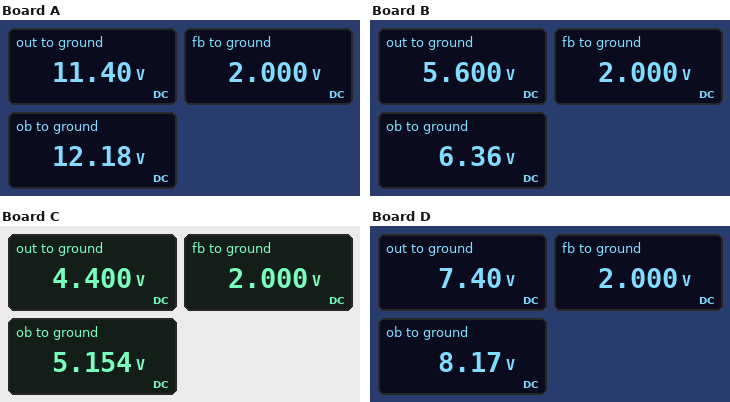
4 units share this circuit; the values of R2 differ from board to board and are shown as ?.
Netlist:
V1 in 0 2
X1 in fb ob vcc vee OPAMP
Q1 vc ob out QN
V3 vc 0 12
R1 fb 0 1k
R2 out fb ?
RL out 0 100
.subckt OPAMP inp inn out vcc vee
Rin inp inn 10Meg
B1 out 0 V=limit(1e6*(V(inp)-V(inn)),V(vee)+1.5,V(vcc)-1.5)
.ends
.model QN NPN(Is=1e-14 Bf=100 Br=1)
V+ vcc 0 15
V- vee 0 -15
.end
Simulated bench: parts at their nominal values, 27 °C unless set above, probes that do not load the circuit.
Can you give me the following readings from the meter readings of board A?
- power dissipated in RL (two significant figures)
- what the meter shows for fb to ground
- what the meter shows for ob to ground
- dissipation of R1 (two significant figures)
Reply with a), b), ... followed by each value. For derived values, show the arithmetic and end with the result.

a) (11.4 V)^2 / 100 Ω = 1.3 W
b) 2.000 V
c) 12.18 V
d) (2 V)^2 / 1 kΩ = 4.0 mW
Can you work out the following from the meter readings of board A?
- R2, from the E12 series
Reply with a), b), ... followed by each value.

a) 4.7 kΩ
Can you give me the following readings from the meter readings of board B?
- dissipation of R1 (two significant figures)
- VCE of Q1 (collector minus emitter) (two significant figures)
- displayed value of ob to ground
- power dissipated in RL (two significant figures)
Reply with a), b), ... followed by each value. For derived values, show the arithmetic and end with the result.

a) (2 V)^2 / 1 kΩ = 4.0 mW
b) 12 V - 5.6 V = 6.4 V
c) 6.36 V
d) (5.6 V)^2 / 100 Ω = 310 mW
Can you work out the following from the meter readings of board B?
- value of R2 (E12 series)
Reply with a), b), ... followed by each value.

a) 1.8 kΩ
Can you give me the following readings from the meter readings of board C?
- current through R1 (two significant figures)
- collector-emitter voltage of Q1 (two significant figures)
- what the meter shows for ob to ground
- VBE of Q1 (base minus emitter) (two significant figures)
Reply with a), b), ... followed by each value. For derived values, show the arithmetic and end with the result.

a) (2 V) / 1 kΩ = 2.0 mA
b) 12 V - 4.4 V = 7.6 V
c) 5.154 V
d) 5.154 V - 4.4 V = 750 mV
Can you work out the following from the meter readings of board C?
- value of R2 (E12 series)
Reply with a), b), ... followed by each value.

a) 1.2 kΩ
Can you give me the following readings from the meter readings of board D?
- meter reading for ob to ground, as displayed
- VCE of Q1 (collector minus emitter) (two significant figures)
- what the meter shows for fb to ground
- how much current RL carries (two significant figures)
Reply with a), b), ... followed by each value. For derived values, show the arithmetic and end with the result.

a) 8.17 V
b) 12 V - 7.4 V = 4.6 V
c) 2.000 V
d) (7.4 V) / 100 Ω = 74 mA
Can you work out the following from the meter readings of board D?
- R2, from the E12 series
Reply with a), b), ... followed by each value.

a) 2.7 kΩ
